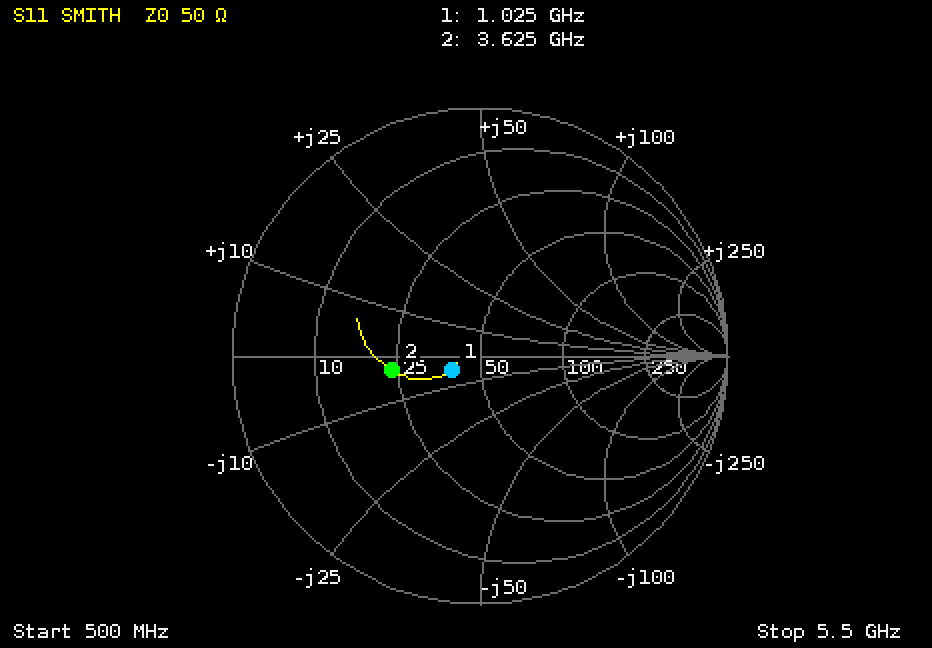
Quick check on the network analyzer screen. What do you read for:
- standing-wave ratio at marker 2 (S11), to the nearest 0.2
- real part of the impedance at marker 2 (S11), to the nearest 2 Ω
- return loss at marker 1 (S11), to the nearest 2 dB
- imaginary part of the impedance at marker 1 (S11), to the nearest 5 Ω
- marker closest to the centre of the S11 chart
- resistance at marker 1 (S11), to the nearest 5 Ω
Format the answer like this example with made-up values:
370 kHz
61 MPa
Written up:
2.2
24 Ω
18 dB
-5 Ω
marker 1
40 Ω
